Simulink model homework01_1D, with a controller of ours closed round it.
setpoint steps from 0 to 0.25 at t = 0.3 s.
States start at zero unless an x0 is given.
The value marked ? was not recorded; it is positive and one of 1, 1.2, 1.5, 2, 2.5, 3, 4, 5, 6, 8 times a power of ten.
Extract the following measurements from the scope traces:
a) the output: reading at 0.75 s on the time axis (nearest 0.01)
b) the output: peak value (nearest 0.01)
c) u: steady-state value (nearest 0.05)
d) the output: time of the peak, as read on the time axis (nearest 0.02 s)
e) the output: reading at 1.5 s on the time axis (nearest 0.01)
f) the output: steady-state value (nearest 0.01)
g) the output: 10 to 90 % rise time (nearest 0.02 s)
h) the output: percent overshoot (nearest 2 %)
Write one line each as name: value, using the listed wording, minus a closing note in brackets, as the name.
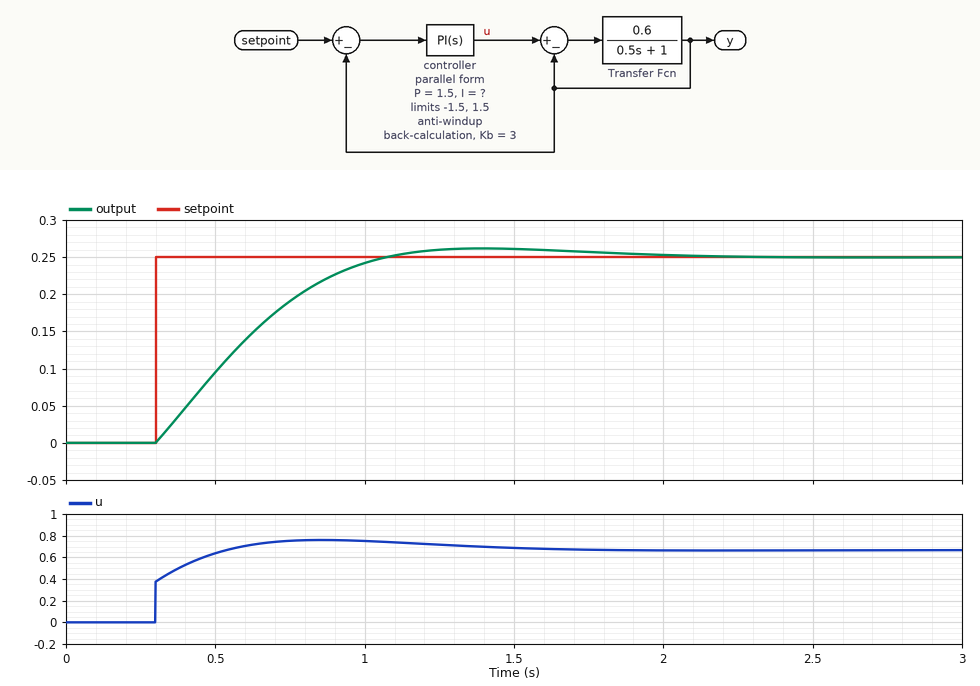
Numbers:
the output: reading at 0.75 s on the time axis: 0.19
the output: peak value: 0.26
u: steady-state value: 0.65
the output: time of the peak, as read on the time axis: 1.40 s
the output: reading at 1.5 s on the time axis: 0.26
the output: steady-state value: 0.25
the output: 10 to 90 % rise time: 0.54 s
the output: percent overshoot: 4 %
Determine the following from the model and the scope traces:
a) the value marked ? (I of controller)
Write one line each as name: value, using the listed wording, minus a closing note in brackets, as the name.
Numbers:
the value marked ?: 10
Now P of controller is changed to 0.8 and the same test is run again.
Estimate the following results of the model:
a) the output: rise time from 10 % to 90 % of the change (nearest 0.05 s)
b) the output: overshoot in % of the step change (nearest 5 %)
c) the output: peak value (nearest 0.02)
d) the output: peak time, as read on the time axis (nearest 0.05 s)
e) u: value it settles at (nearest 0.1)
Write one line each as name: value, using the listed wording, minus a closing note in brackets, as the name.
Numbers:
the output: rise time from 10 % to 90 % of the change: 0.50 s
the output: overshoot in % of the step change: 10 %
the output: peak value: 0.28
the output: peak time, as read on the time axis: 1.35 s
u: value it settles at: 0.7
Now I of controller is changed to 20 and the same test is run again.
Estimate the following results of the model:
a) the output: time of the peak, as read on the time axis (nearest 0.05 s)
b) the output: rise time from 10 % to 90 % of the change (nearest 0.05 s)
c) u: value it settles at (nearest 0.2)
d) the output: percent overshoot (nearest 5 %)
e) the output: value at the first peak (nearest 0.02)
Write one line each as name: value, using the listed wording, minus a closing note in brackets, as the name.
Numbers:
the output: time of the peak, as read on the time axis: 0.95 s
the output: rise time from 10 % to 90 % of the change: 0.30 s
u: value it settles at: 0.6
the output: percent overshoot: 15 %
the output: value at the first peak: 0.30
